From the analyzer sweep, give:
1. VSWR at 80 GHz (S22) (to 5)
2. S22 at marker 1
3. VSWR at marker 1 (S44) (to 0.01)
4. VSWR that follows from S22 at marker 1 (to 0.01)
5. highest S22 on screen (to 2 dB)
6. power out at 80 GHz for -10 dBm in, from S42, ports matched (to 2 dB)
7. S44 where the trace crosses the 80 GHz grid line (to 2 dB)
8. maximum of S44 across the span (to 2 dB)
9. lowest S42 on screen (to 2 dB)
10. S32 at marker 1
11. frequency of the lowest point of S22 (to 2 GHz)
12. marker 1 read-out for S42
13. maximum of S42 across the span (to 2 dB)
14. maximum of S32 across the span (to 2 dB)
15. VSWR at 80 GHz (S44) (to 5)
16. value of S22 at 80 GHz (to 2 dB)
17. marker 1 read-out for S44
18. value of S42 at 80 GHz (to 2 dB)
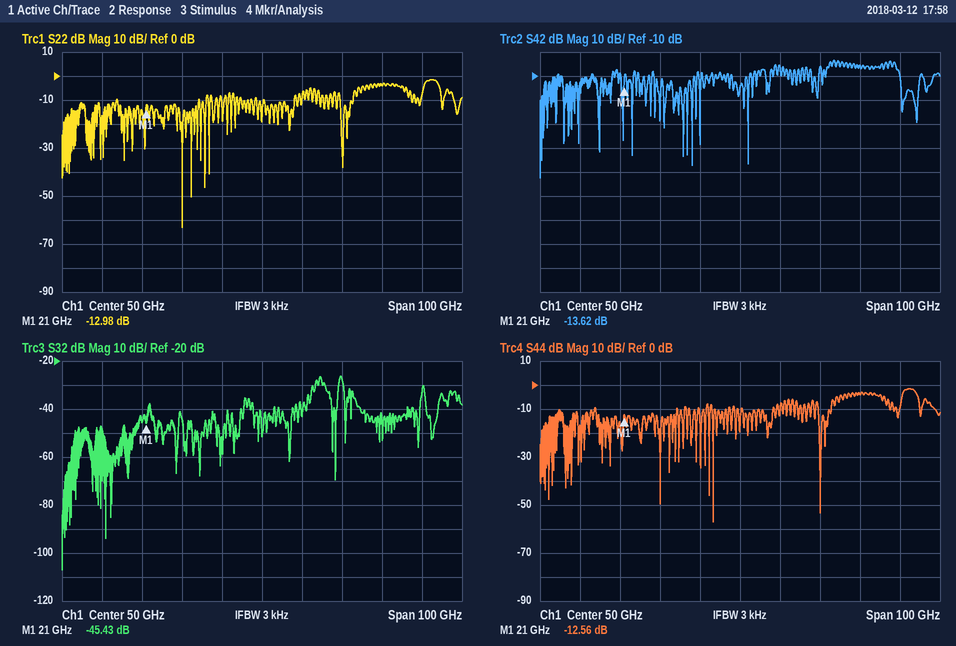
5
-12.98 dB
1.62
1.58
-2 dB
-16 dBm
-4 dB
-2 dB
-52 dB
-45.43 dB
30 GHz
-13.62 dB
-4 dB
-26 dB
5
-4 dB
-12.56 dB
-6 dB
